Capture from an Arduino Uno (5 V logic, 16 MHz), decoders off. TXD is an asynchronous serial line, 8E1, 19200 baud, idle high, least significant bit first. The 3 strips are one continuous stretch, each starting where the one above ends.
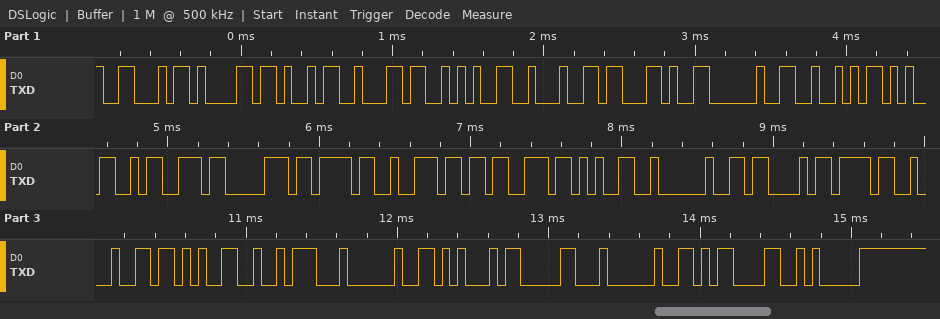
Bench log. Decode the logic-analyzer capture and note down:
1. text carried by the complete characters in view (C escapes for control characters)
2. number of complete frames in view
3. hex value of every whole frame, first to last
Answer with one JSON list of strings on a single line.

["\"Failed, Response Code: E0 \\r\\n\"", "28", "46 61 69 6C 65 64 2C 20 52 65 73 70 6F 6E 73 65 20 43 6F 64 65 3A 20 45 30 20 0D 0A"]
